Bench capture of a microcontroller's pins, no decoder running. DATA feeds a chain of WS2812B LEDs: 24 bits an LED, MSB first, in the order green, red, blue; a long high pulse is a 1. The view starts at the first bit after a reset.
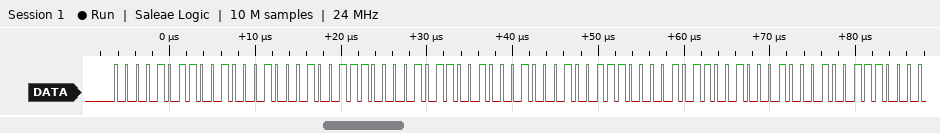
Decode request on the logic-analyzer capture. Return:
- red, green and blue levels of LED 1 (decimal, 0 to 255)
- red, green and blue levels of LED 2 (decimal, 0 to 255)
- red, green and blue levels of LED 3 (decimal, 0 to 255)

34, 11, 39
34, 11, 39
34, 11, 39
